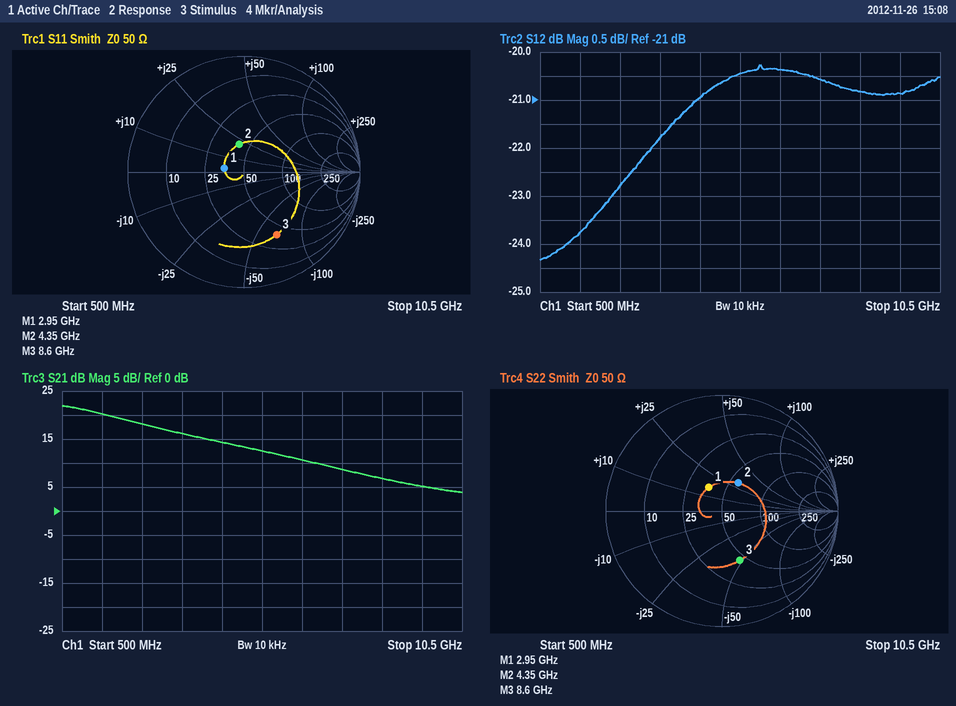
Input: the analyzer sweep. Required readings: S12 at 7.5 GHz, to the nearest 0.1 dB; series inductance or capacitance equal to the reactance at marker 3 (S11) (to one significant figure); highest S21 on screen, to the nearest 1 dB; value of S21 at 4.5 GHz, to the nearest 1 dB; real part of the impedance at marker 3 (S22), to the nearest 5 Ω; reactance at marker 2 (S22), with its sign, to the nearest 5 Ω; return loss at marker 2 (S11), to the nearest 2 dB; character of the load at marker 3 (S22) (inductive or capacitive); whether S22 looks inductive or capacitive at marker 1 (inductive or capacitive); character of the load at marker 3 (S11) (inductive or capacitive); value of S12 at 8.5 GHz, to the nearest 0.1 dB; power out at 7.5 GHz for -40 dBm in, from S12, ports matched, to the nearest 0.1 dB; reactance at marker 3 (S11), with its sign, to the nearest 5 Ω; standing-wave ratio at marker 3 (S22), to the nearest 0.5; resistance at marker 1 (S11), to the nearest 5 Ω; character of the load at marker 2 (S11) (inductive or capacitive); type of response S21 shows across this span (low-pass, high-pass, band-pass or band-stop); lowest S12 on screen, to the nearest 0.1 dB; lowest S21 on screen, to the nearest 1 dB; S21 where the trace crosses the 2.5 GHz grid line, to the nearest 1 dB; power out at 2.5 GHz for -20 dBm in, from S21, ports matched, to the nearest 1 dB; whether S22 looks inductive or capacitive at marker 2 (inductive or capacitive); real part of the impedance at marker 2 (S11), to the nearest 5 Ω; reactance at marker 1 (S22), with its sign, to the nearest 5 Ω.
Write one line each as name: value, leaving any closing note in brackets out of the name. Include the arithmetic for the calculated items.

S12 at 7.5 GHz, to the nearest 0.1 dB: -20.6 dB
series inductance or capacitance equal to the reactance at marker 3 (S11): C = 1/(2π × 8.6 GHz × 65 Ω) ≈ 285 fF, so 300 fF to one significant figure
highest S21 on screen, to the nearest 1 dB: 22 dB
value of S21 at 4.5 GHz, to the nearest 1 dB: 14 dB
real part of the impedance at marker 3 (S22), to the nearest 5 Ω: 45 Ω
reactance at marker 2 (S22), with its sign, to the nearest 5 Ω: +30 Ω
return loss at marker 2 (S11), to the nearest 2 dB: 12 dB
character of the load at marker 3 (S22): capacitive
whether S22 looks inductive or capacitive at marker 1: inductive
character of the load at marker 3 (S11): capacitive
value of S12 at 8.5 GHz, to the nearest 0.1 dB: -20.8 dB
power out at 7.5 GHz for -40 dBm in, from S12, ports matched, to the nearest 0.1 dB: -40 dBm + (-20.6 dB) = -60.6 dBm
reactance at marker 3 (S11), with its sign, to the nearest 5 Ω: -65 Ω
standing-wave ratio at marker 3 (S22), to the nearest 0.5: 2.5
resistance at marker 1 (S11), to the nearest 5 Ω: 35 Ω
character of the load at marker 2 (S11): inductive
type of response S21 shows across this span: low-pass
lowest S12 on screen, to the nearest 0.1 dB: -24.3 dB
lowest S21 on screen, to the nearest 1 dB: 4 dB
S21 where the trace crosses the 2.5 GHz grid line, to the nearest 1 dB: 18 dB
power out at 2.5 GHz for -20 dBm in, from S21, ports matched, to the nearest 1 dB: -20 dBm + (18 dB) = -2 dBm
whether S22 looks inductive or capacitive at marker 2: inductive
real part of the impedance at marker 2 (S11), to the nearest 5 Ω: 40 Ω
reactance at marker 1 (S22), with its sign, to the nearest 5 Ω: +15 Ω
